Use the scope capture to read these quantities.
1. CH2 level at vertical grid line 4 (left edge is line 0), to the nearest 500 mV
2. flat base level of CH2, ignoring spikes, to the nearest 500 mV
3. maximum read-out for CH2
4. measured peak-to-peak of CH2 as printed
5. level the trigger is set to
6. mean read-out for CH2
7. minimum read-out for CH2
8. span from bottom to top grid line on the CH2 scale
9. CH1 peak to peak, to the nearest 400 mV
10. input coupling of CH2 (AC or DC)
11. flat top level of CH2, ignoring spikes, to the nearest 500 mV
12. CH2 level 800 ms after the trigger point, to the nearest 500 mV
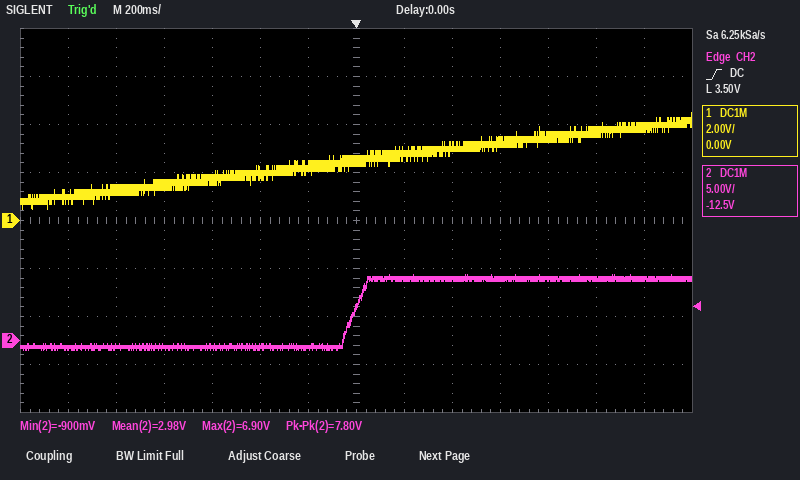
-500 mV
-500 mV
6.90 V
7.80 V
3.50 V
2.98 V
-900 mV
40 V
4.0 V
DC
6.5 V
6.5 V
